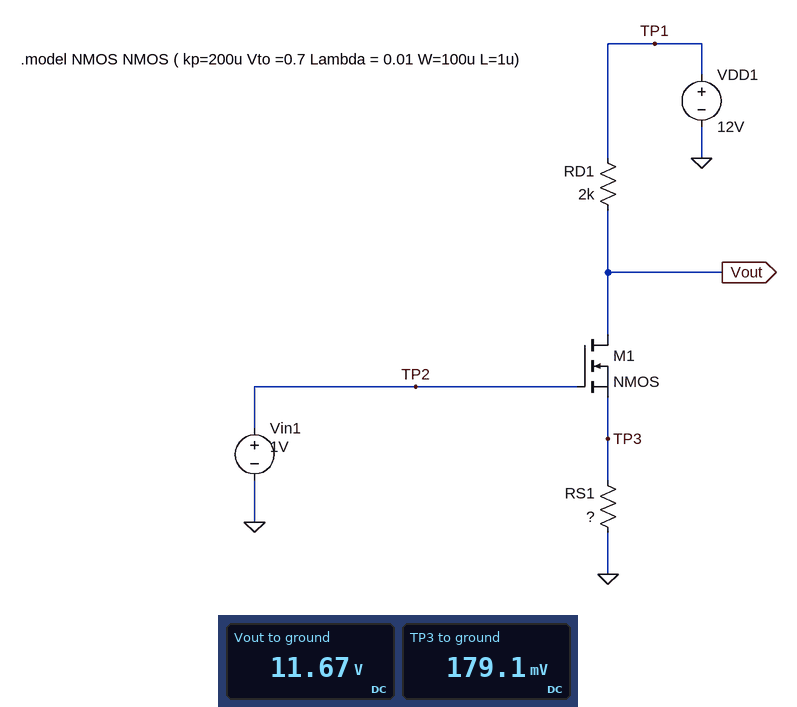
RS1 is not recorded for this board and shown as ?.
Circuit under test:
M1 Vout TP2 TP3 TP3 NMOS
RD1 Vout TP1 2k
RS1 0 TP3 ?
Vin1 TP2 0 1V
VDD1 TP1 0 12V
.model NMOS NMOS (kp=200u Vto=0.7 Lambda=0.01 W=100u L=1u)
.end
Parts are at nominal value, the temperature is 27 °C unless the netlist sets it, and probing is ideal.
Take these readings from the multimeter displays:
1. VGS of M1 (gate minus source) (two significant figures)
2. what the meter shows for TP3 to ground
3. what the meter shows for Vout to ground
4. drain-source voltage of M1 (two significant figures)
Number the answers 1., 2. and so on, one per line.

1. 820 mV
2. 179.1 mV
3. 11.67 V
4. 11 V
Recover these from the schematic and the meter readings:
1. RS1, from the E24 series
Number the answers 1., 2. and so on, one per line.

1. 1.1 kΩ
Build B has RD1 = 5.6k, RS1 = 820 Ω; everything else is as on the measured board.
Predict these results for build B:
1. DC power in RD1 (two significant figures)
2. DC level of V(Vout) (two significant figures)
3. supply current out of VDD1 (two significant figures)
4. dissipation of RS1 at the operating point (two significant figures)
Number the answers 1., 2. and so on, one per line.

1. 230 µW
2. 11 V
3. 200 µA
4. 33 µW
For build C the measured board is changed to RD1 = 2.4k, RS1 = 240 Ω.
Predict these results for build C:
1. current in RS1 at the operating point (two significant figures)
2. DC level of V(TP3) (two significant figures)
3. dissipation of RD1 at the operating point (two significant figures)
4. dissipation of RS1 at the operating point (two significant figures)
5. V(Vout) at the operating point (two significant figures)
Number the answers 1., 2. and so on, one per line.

1. 430 µA
2. 100 mV
3. 440 µW
4. 44 µW
5. 11 V
